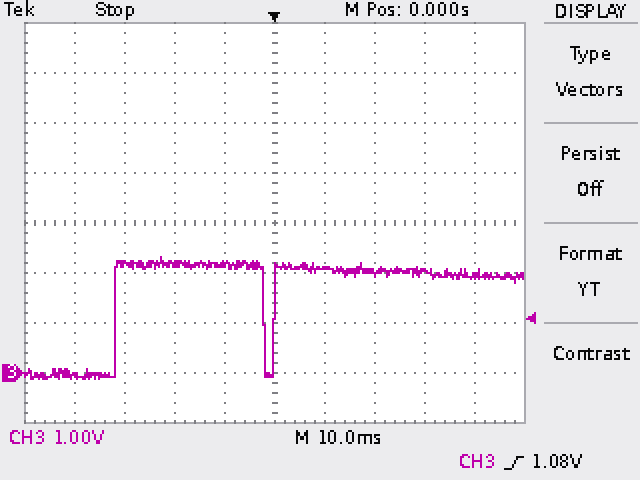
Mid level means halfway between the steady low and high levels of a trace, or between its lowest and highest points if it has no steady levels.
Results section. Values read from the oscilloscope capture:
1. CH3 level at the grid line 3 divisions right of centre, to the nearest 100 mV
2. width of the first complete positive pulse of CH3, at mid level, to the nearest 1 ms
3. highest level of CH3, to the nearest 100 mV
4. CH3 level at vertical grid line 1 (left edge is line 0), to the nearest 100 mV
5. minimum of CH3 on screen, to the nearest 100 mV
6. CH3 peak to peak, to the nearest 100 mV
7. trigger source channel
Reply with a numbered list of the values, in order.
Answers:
1. 2.0 V
2. 30 ms
3. 2.3 V
4. -100 mV
5. -100 mV
6. 2.4 V
7. CH3
